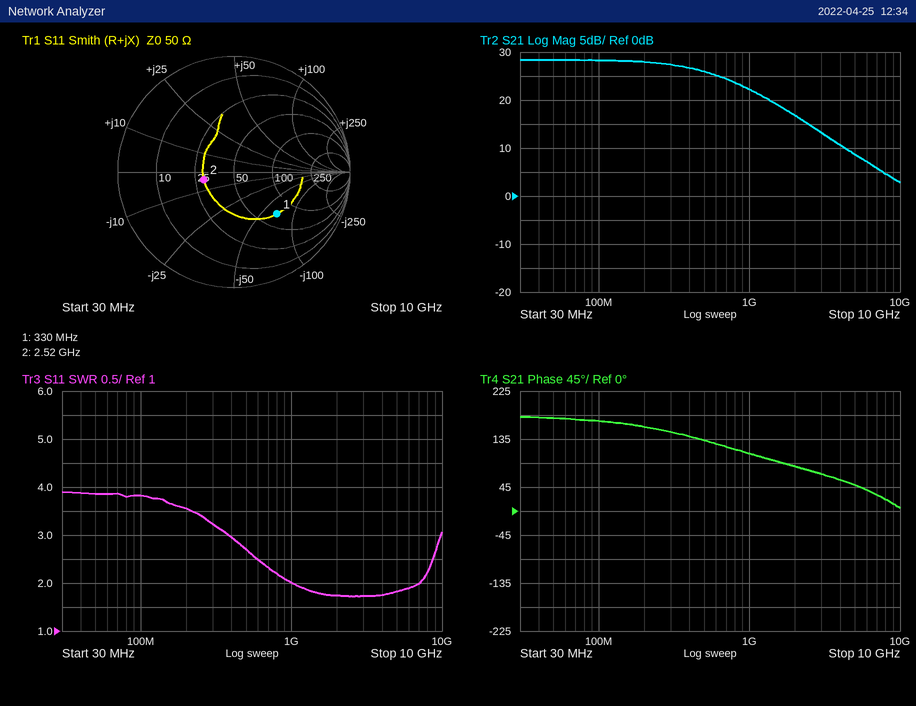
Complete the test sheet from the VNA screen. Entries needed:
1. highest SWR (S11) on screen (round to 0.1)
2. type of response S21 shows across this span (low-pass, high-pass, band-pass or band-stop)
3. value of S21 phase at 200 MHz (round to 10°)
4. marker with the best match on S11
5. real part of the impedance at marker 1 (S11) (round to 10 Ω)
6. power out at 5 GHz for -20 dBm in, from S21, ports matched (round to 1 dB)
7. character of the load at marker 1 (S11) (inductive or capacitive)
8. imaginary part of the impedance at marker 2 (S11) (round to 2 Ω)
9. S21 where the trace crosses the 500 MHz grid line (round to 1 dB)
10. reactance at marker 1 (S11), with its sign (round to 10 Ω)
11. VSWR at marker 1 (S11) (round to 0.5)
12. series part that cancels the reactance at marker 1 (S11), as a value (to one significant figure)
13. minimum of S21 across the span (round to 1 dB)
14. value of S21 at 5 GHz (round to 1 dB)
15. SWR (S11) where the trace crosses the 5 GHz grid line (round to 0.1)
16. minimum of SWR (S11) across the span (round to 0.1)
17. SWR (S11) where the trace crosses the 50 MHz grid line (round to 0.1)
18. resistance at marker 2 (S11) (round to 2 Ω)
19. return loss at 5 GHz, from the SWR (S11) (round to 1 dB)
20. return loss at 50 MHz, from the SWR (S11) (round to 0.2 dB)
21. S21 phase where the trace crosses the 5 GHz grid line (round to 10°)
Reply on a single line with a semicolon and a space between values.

3.9; low-pass; 160°; marker 2; 70 Ω; -11 dBm; capacitive; -4 Ω; 26 dB; -70 Ω; 3.0; 30 nH; 3 dB; 9 dB; 1.8; 1.7; 3.9; 30 Ω; 11 dB; 4.6 dB; 50°
